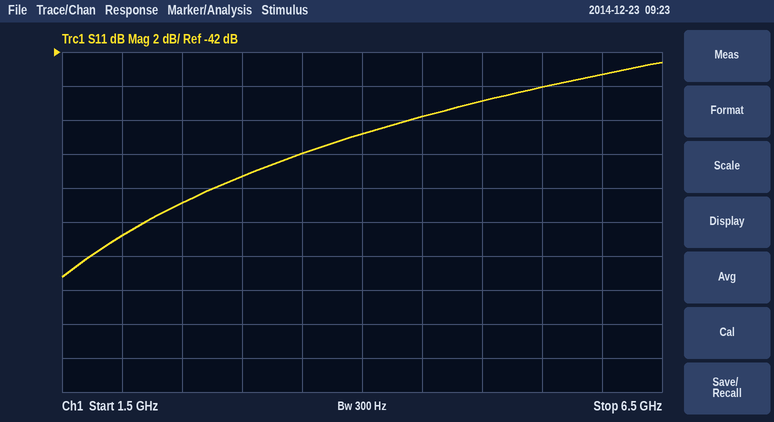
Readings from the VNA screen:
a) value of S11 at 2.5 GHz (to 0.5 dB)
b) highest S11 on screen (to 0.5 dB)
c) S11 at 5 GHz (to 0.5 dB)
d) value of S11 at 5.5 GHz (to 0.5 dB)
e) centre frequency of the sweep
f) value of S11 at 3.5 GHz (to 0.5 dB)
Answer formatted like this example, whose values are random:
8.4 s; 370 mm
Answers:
-51.0 dB; -42.5 dB; -45.0 dB; -44.0 dB; 4 GHz; -48.0 dB
